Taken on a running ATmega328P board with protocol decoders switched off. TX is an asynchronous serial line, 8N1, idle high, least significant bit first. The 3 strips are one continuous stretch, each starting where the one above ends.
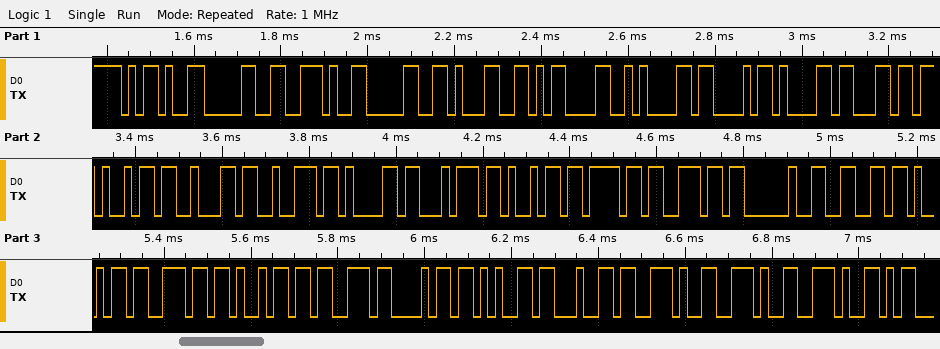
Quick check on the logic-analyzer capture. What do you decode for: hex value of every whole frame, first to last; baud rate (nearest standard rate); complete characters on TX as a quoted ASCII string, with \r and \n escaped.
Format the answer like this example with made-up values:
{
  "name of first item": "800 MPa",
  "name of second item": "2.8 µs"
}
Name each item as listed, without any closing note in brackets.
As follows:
{
  "hex value of every whole frame, first to last": "2D 30 2E 30 31 0D 0A 43 61 6C 69 62 72 61 74 69 6F 6E 20 66 69 6E 69 73 68 65 64 2E 2E 2E",
  "baud rate": "57600 baud",
  "complete characters on TX as a quoted ASCII string, with \\r and \\n escaped": "\"-0.01\\r\\nCalibration finished...\""
}
